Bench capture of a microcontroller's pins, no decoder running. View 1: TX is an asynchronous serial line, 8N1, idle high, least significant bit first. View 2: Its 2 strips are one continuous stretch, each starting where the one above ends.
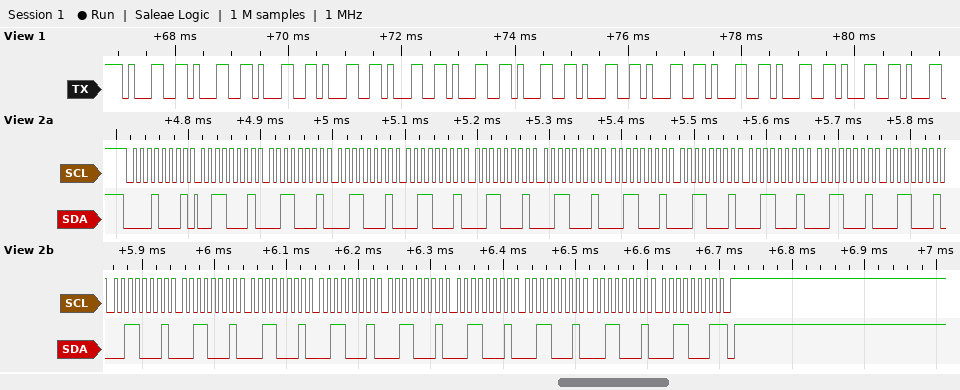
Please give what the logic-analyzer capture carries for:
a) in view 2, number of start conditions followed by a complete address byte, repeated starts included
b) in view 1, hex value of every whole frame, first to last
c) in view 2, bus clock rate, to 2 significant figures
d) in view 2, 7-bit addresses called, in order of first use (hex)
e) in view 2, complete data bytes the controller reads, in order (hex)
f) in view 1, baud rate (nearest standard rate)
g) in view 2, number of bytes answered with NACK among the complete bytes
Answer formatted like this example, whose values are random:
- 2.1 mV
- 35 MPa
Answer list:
- 1
- 31 31 31 31 31 31 31 31 31 31 31 31
- 100 kHz
- 0x08
- 31 31 31 31 31 31 31 31 31 31 31 31 31 31 31 31 31 31 31 31
- 9600 baud
- 1
